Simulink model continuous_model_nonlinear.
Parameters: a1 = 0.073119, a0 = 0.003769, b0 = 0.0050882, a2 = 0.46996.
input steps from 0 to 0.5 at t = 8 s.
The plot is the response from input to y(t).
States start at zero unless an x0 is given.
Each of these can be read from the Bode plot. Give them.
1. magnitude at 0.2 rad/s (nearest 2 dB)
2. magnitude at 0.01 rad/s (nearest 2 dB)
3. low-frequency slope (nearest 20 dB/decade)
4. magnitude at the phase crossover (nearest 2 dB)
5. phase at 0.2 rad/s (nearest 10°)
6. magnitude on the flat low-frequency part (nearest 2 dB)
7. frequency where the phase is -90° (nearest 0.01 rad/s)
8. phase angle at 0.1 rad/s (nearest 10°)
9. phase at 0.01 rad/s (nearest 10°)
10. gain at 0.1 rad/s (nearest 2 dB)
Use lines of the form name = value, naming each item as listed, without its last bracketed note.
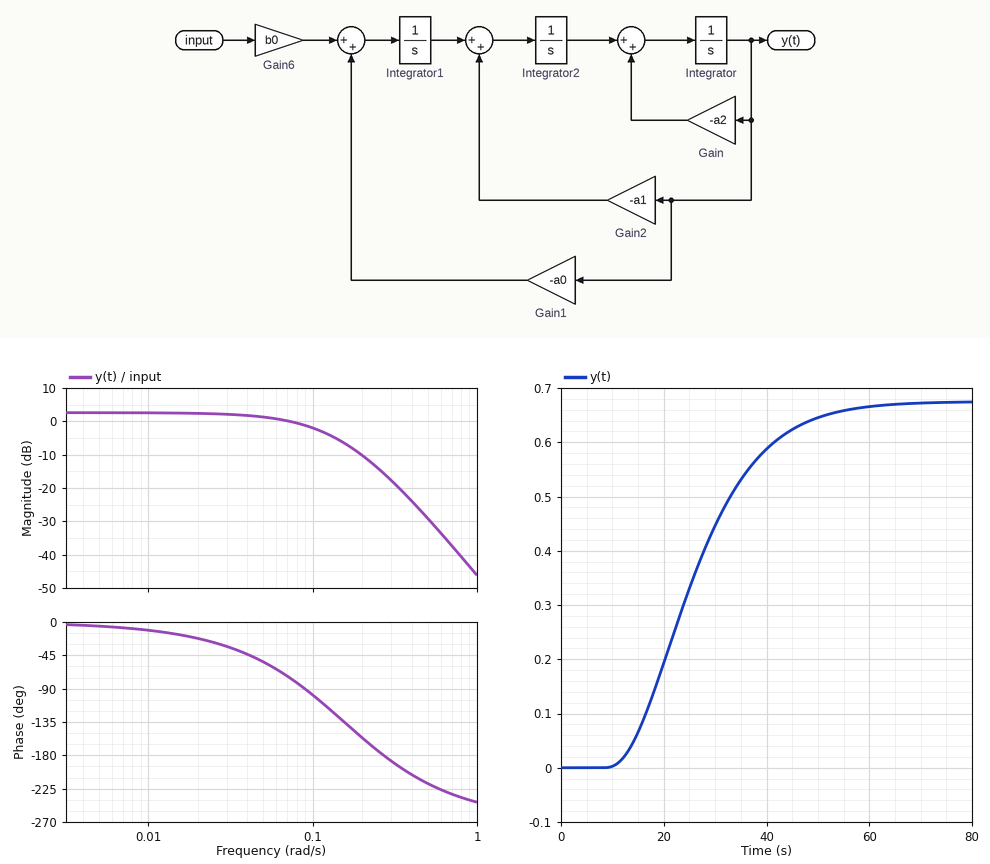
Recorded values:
magnitude at 0.2 rad/s = -10 dB
magnitude at 0.01 rad/s = 2 dB
low-frequency slope = 0 dB/decade
magnitude at the phase crossover = -16 dB
phase at 0.2 rad/s = -160°
magnitude on the flat low-frequency part = 2 dB
frequency where the phase is -90° = 0.09 rad/s
phase angle at 0.1 rad/s = -100°
phase at 0.01 rad/s = -10°
gain at 0.1 rad/s = -2 dB
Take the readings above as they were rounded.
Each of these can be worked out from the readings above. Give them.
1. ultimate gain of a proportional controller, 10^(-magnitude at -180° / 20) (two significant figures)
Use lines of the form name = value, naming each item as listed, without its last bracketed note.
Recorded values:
ultimate gain of a proportional controller, 10^(-magnitude at -180° / 20) = 6.3
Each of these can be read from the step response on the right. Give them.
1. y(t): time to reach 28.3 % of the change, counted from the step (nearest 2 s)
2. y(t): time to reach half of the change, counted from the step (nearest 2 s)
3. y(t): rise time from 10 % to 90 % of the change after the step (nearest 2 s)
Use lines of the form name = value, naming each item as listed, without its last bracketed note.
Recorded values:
y(t): time to reach 28.3 % of the change, counted from the step = 12 s
y(t): time to reach half of the change, counted from the step = 18 s
y(t): rise time from 10 % to 90 % of the change after the step = 28 s
